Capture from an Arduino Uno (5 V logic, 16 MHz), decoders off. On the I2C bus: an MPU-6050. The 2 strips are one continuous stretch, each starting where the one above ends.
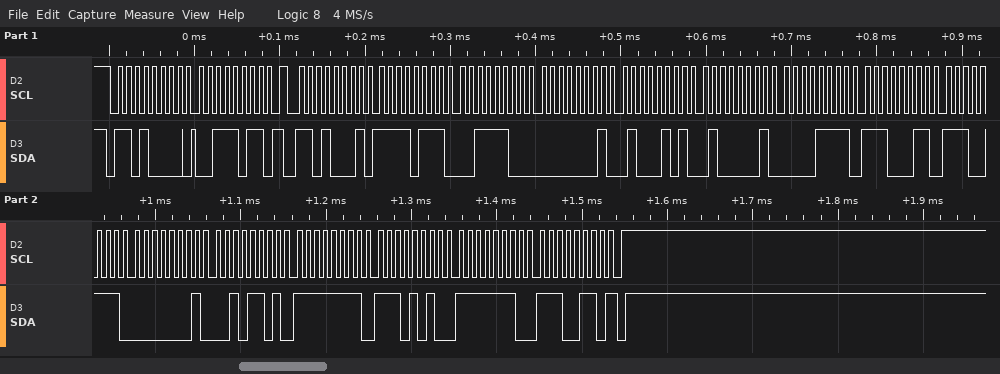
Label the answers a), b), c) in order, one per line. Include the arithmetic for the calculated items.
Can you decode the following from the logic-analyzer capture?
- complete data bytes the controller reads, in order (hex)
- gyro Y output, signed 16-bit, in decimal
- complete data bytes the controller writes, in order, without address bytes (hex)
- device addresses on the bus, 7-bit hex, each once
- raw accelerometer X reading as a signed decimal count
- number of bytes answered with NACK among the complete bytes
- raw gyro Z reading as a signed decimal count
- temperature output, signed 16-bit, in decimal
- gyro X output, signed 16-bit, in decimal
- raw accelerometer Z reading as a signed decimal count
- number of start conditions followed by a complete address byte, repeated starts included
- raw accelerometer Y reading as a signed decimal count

a) F7 3C 01 45 41 0F E3 E7 01 2D FF EA FE E6
b) 0xFFEA = -22
c) 3B
d) 0x68
e) 0xF73C = -2244
f) 1
g) 0xFEE6 = -282
h) 0xE3E7 = -7193
i) 0x012D = 301
j) 0x410F = 16655
k) 2
l) 0x0145 = 325
